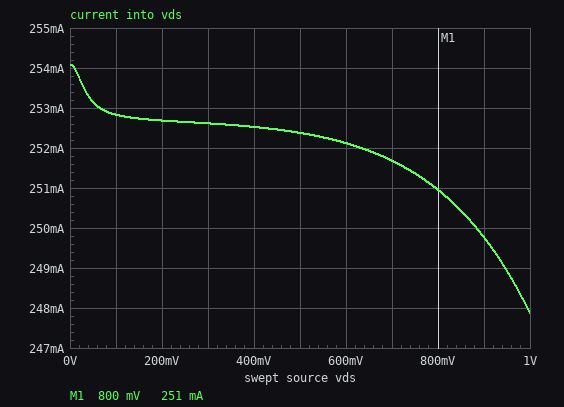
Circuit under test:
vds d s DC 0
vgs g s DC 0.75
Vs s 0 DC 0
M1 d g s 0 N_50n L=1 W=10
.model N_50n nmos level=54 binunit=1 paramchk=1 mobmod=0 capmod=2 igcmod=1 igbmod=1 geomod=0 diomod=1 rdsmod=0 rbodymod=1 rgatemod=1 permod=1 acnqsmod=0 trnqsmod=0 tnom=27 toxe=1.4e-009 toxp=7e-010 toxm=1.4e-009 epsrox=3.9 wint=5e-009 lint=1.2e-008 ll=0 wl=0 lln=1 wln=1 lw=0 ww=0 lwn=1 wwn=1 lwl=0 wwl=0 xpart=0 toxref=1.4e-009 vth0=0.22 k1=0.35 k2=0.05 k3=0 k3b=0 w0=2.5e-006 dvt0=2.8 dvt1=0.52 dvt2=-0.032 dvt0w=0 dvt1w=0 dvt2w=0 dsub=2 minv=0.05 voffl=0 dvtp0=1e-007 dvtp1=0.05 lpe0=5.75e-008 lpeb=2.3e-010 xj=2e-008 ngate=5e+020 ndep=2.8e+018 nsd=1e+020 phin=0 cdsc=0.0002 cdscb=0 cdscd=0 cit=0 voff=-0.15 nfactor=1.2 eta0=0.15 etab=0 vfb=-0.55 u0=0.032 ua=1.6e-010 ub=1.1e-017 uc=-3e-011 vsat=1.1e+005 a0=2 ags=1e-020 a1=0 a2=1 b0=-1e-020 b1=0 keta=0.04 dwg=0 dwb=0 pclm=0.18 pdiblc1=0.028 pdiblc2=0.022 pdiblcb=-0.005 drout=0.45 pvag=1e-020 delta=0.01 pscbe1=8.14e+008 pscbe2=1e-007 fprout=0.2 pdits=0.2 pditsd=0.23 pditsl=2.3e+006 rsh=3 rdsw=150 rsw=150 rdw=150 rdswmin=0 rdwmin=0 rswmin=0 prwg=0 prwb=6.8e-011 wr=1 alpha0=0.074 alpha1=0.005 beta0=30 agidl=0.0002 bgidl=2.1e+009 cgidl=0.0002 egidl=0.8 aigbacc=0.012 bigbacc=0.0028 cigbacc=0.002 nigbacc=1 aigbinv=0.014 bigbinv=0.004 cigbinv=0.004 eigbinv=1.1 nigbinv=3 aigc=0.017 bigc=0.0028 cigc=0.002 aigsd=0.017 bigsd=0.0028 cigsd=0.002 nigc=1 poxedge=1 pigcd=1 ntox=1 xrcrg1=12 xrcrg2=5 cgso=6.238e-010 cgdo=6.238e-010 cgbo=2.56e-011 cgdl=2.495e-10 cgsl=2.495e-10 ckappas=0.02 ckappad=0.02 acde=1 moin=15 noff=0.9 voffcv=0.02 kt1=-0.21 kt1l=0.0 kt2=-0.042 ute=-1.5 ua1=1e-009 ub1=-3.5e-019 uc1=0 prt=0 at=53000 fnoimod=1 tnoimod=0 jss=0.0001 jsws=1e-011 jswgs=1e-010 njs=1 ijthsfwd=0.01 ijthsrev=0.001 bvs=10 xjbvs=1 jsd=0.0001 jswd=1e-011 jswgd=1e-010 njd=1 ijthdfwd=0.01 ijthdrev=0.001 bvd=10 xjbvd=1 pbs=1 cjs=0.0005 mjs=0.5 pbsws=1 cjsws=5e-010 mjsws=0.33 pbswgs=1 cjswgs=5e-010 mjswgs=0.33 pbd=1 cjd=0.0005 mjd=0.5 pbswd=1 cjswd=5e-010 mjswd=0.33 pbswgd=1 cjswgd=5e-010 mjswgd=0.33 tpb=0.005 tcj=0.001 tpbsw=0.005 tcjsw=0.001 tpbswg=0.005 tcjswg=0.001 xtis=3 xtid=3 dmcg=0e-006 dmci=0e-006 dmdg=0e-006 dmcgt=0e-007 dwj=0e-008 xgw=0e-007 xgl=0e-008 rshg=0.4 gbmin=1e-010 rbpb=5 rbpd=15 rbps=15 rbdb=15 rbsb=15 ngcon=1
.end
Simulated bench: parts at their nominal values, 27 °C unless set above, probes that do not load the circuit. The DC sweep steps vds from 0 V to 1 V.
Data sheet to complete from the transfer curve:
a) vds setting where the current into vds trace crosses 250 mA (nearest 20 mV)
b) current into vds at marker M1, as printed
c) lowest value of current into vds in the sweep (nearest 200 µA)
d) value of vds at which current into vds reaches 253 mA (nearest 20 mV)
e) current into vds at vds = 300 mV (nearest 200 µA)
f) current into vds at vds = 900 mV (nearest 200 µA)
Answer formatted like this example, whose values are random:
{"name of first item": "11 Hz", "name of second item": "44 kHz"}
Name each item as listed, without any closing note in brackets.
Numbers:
{"vds setting where the current into vds trace crosses 250 mA": "880 mV", "current into vds at marker M1, as printed": "251 mA", "lowest value of current into vds in the sweep": "247.8 mA", "value of vds at which current into vds reaches 253 mA": "60 mV", "current into vds at vds = 300 mV": "252.6 mA", "current into vds at vds = 900 mV": "249.8 mA"}
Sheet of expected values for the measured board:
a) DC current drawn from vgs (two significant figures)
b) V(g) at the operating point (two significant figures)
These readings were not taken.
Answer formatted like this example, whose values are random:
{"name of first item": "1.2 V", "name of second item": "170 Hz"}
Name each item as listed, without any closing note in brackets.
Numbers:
{"DC current drawn from vgs": "510 mA", "V(g) at the operating point": "750 mV"}
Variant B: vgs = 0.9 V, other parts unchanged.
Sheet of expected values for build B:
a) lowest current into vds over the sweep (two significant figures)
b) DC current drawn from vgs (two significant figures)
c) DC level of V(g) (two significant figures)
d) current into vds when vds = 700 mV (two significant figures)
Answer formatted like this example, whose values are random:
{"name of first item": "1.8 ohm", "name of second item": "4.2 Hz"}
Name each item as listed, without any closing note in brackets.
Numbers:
{"lowest current into vds over the sweep": "300 mA", "DC current drawn from vgs": "620 mA", "DC level of V(g)": "900 mV", "current into vds when vds = 700 mV": "310 mA"}
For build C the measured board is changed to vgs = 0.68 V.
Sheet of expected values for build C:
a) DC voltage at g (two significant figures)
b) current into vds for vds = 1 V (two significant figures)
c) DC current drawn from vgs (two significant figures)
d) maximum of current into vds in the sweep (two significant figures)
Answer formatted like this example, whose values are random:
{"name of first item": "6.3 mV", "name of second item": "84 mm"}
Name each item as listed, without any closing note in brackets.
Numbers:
{"DC voltage at g": "680 mV", "current into vds for vds = 1 V": "220 mA", "DC current drawn from vgs": "460 mA", "maximum of current into vds in the sweep": "230 mA"}
